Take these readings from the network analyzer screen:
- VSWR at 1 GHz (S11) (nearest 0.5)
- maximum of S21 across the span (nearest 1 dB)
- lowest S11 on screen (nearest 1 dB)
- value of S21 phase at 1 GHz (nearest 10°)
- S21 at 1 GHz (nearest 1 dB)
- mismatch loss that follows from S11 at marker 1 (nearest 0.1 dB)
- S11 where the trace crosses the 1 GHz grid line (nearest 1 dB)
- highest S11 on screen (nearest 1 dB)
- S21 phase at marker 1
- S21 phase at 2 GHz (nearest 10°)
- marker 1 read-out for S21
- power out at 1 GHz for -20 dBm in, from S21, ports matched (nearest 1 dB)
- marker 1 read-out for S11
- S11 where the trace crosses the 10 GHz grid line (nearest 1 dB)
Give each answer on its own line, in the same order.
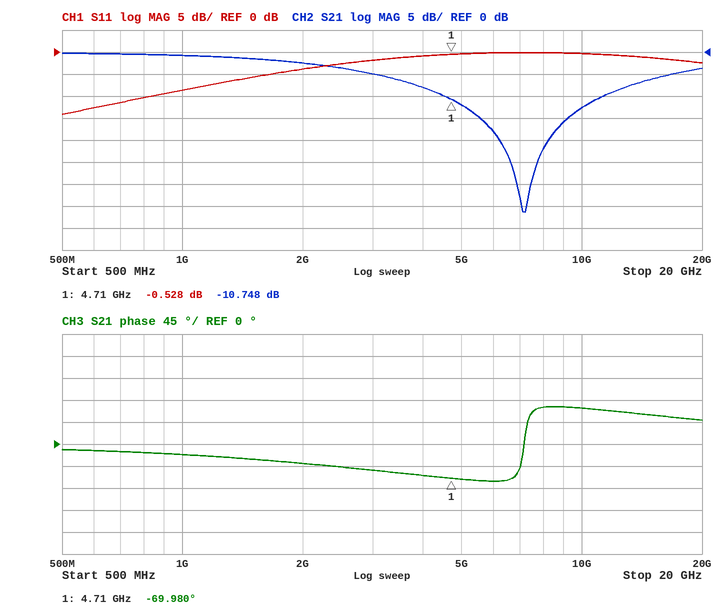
2.0
0 dB
-14 dB
-20°
-1 dB
9.4 dB
-9 dB
0 dB
-69.980°
-40°
-10.748 dB
-21 dBm
-0.528 dB
0 dB
